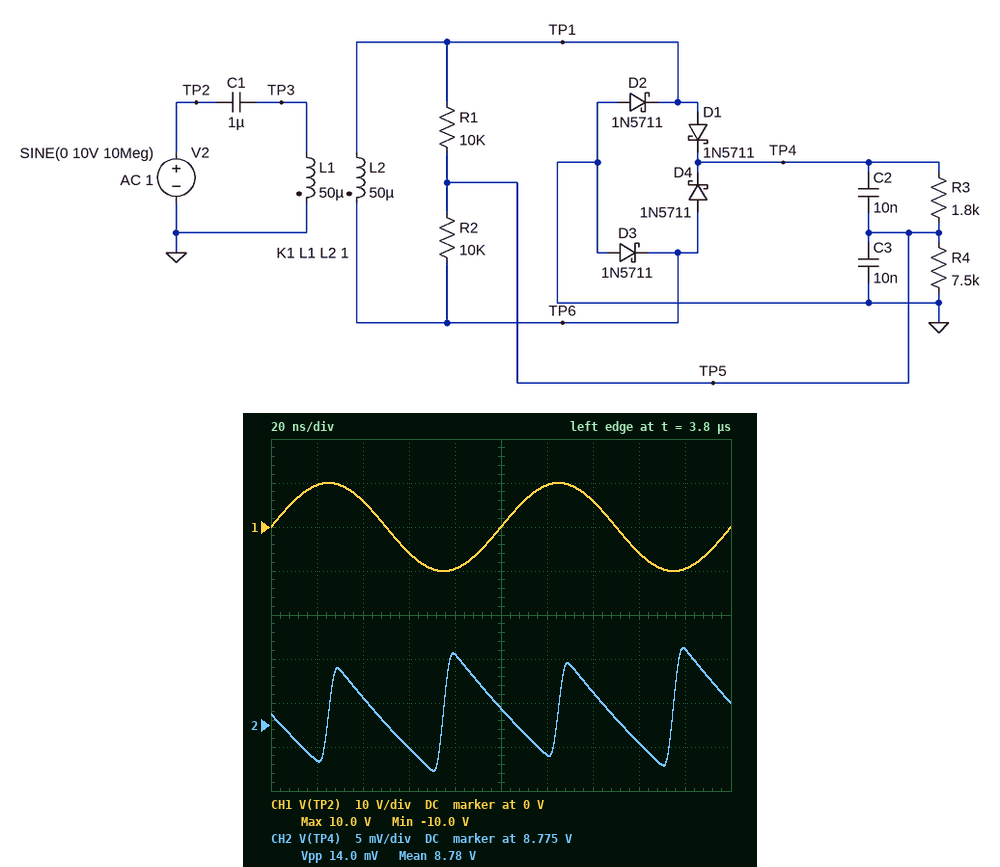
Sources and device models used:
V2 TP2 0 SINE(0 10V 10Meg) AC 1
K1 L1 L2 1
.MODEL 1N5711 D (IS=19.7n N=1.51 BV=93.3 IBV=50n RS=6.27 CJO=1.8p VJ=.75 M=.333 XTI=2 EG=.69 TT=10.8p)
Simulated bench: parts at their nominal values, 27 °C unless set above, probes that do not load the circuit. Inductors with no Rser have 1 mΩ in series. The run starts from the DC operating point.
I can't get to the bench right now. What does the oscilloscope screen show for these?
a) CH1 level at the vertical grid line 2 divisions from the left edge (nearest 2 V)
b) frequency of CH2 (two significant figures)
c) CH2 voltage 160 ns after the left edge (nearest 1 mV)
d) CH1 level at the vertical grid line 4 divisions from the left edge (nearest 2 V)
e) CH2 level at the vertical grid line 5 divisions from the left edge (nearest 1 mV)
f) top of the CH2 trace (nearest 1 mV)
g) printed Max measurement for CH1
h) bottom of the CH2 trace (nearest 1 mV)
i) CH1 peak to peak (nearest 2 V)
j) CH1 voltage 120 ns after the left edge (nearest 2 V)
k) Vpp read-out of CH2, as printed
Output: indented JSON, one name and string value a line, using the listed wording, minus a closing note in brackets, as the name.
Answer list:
{
  "CH1 level at the vertical grid line 2 divisions from the left edge": "6 V",
  "frequency of CH2": "20 MHz",
  "CH2 voltage 160 ns after the left edge": "8.773 V",
  "CH1 level at the vertical grid line 4 divisions from the left edge": "-10 V",
  "CH2 level at the vertical grid line 5 divisions from the left edge": "8.777 V",
  "top of the CH2 trace": "8.784 V",
  "printed Max measurement for CH1": "10.0 V",
  "bottom of the CH2 trace": "8.770 V",
  "CH1 peak to peak": "20 V",
  "CH1 voltage 120 ns after the left edge": "10 V",
  "Vpp read-out of CH2, as printed": "14.0 mV"
}
